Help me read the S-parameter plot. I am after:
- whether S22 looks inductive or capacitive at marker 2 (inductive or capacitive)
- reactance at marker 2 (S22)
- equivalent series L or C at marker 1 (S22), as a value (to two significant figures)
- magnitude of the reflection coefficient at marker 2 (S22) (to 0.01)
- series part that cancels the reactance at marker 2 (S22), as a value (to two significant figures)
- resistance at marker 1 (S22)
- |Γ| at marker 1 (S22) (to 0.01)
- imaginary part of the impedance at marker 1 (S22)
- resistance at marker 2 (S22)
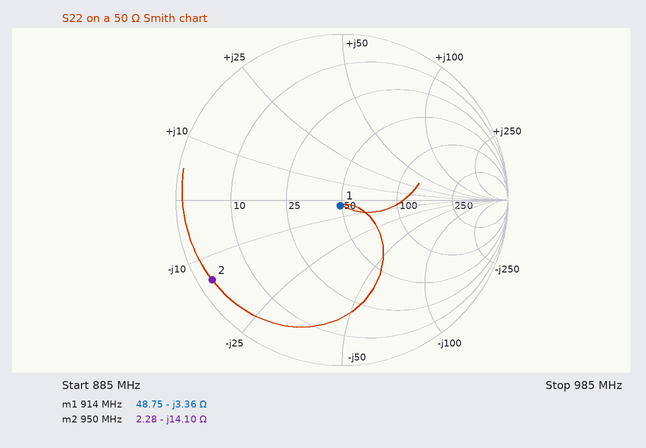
capacitive
-14.10 Ω
52 pF
0.92
2.4 nH
48.75 Ω
0.04
-3.36 Ω
2.28 Ω
